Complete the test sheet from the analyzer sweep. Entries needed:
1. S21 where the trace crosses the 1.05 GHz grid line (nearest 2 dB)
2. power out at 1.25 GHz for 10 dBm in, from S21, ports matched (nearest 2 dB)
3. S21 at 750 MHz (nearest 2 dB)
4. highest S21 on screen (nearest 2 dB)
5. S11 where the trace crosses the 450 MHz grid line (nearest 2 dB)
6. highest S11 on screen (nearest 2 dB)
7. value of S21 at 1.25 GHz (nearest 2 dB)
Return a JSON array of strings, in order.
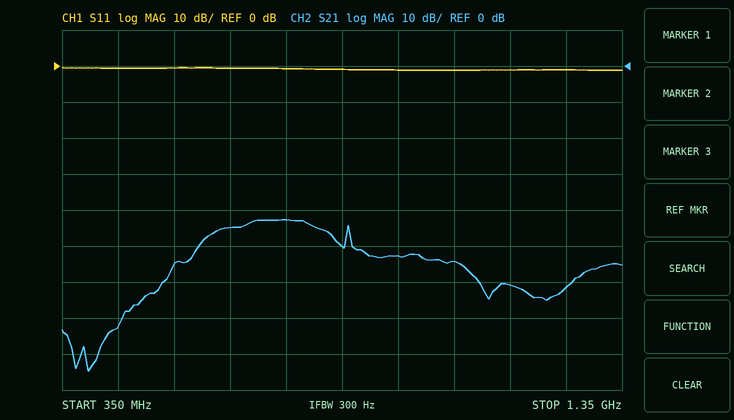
["-54 dB", "-52 dBm", "-42 dB", "-42 dB", "0 dB", "0 dB", "-62 dB"]
